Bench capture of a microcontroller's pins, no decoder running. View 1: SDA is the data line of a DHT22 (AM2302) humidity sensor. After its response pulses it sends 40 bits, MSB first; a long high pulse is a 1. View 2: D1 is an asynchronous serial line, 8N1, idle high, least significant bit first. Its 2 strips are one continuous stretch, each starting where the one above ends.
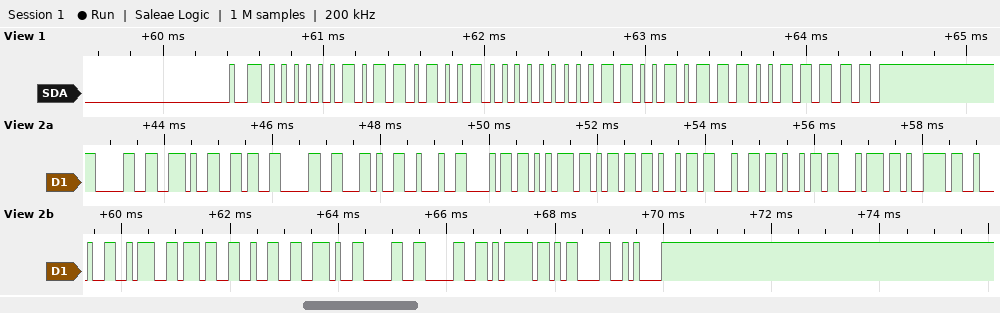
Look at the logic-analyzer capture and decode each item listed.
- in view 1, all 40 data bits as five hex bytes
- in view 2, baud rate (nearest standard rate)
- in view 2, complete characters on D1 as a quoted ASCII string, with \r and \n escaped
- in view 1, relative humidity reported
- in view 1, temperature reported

02 D2 00 CB 9F
9600 baud
"0.60,\"humidity\":72.00}\r\n"
72.2 %
20.3 °C
